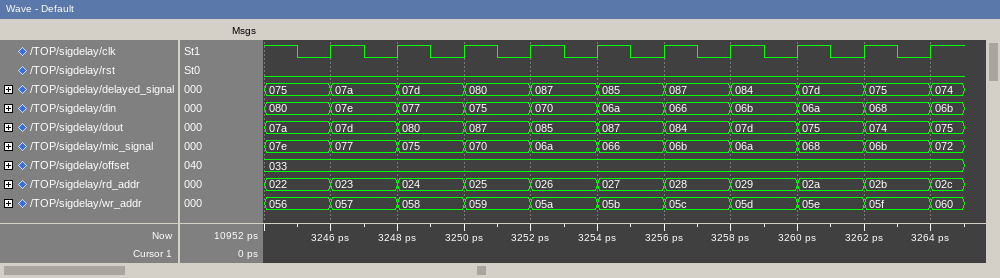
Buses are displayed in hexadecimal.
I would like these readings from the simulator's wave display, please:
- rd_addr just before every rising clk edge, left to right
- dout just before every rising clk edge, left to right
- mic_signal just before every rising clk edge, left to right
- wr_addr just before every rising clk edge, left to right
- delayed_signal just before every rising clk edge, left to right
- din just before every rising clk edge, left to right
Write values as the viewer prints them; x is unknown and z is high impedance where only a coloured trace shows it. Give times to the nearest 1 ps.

022, 023, 024, 025, 026, 027, 028, 029, 02a, 02b
07a, 07d, 080, 087, 085, 087, 084, 07d, 075, 074
07e, 077, 075, 070, 06a, 066, 06b, 06a, 068, 06b
056, 057, 058, 059, 05a, 05b, 05c, 05d, 05e, 05f
075, 07a, 07d, 080, 087, 085, 087, 084, 07d, 075
080, 07e, 077, 075, 070, 06a, 066, 06b, 06a, 068
